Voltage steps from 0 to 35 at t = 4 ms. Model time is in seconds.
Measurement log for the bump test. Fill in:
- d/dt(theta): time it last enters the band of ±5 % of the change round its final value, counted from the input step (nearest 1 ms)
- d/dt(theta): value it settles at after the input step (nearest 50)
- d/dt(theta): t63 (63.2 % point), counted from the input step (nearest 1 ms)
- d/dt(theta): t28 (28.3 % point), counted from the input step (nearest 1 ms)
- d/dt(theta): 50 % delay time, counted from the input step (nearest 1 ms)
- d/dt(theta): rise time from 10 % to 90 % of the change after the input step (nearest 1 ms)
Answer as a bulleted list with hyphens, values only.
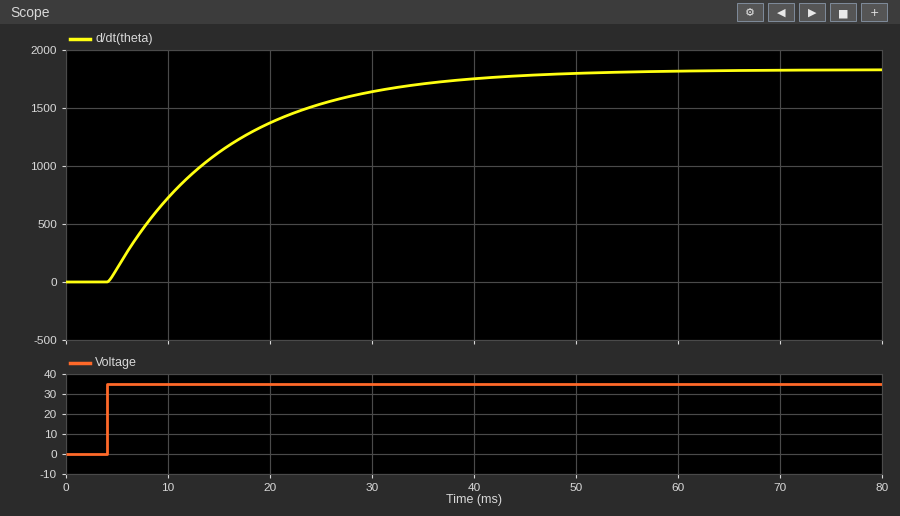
- 34 ms
- 1850
- 12 ms
- 4 ms
- 8 ms
- 25 ms
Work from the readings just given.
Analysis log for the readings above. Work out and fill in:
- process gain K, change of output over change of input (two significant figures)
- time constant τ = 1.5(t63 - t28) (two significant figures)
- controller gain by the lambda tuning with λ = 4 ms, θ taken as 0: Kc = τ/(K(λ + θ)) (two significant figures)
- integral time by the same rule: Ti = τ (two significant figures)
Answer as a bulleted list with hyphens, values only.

- 53
- 12 ms
- 0.057
- 12 ms
